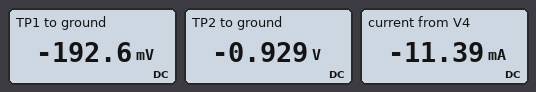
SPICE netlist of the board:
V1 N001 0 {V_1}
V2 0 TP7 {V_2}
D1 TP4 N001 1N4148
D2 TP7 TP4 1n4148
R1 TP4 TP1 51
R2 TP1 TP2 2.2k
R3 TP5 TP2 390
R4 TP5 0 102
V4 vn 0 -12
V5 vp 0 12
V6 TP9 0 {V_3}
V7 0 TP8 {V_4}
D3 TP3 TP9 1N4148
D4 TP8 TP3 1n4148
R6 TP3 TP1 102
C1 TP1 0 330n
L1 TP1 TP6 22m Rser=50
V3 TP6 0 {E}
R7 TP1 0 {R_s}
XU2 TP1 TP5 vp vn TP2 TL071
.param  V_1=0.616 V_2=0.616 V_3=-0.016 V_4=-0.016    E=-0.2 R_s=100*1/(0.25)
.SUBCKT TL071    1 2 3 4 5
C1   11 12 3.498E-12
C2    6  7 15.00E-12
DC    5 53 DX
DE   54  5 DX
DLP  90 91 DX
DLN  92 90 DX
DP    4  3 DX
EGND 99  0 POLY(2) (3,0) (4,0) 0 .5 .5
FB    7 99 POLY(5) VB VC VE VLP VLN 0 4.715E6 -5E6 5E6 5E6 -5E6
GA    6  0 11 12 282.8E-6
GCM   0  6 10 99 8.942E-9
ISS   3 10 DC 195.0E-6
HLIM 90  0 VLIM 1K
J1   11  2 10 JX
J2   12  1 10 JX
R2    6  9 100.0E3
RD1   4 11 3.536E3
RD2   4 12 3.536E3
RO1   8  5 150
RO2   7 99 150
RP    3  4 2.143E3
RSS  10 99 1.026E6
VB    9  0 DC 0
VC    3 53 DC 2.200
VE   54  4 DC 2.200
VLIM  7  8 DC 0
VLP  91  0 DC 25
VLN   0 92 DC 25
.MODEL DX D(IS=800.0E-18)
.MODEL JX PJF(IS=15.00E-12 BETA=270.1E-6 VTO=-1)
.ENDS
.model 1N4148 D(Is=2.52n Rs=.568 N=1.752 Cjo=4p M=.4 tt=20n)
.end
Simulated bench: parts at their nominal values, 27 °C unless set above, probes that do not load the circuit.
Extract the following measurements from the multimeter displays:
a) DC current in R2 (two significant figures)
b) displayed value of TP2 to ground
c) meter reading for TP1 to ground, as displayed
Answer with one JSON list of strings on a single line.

["330 µA", "-0.929 V", "-192.6 mV"]
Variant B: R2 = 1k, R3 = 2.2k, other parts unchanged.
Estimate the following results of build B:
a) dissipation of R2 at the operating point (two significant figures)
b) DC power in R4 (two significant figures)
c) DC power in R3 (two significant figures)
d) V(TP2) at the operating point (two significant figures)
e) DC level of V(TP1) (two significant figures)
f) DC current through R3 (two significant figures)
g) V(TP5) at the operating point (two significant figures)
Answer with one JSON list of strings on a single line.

["97 mW", "2.1 mW", "45 mW", "-10 V", "-590 mV", "4.5 mA", "-460 mV"]
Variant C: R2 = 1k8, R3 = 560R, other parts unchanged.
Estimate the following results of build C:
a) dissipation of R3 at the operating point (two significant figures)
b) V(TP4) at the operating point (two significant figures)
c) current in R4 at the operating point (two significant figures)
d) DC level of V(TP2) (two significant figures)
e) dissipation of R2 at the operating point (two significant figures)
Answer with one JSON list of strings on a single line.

["2.3 mW", "-210 mV", "2.0 mA", "-1.3 V", "710 µW"]
